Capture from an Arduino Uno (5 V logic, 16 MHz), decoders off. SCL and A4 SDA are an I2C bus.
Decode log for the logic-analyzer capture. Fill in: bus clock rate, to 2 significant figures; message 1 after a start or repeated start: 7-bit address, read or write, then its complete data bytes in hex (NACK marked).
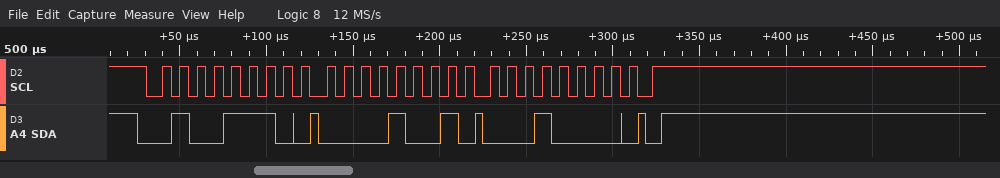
100 kHz
0x27 write: 09 10
